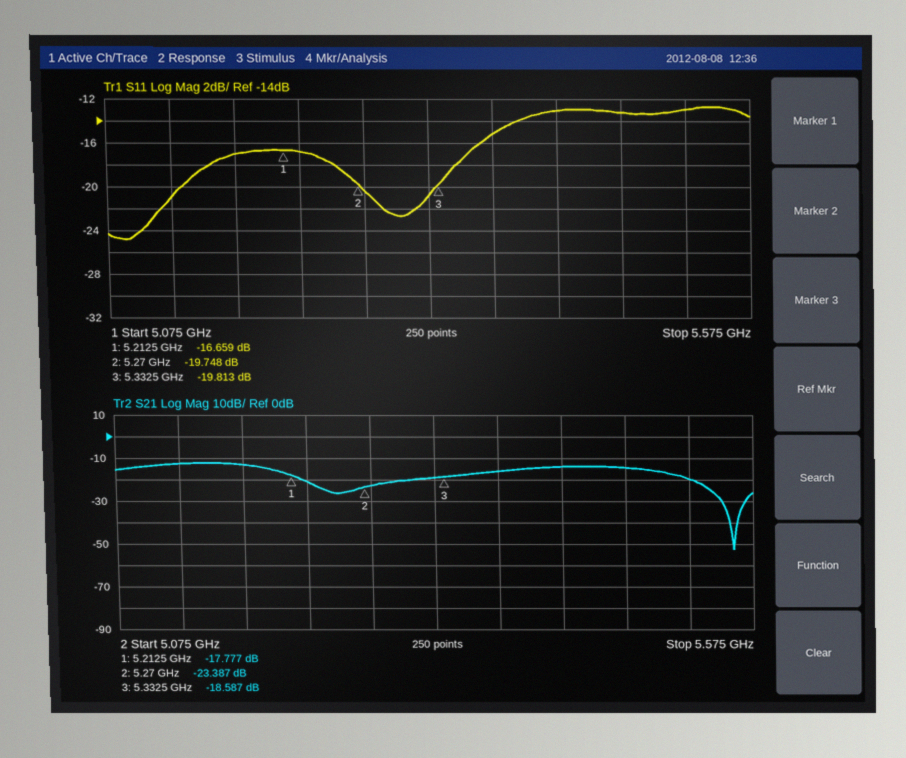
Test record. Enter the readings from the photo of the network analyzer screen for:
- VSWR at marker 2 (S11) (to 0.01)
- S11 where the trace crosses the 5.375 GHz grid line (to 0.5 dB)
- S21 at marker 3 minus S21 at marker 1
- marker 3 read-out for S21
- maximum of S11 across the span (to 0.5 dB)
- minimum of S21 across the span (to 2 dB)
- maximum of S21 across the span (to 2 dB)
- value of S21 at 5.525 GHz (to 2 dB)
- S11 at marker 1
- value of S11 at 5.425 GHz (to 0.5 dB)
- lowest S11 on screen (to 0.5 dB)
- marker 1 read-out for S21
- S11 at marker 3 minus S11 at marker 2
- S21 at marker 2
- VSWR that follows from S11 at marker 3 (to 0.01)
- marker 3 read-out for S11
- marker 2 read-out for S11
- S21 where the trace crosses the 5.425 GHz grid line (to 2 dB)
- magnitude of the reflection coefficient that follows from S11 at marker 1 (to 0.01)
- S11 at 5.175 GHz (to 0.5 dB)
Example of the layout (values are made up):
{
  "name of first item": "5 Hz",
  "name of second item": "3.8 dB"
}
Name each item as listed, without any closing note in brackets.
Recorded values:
{
  "VSWR at marker 2 (S11)": "1.23",
  "S11 where the trace crosses the 5.375 GHz grid line": "-15.0 dB",
  "S21 at marker 3 minus S21 at marker 1": "-0.810 dB",
  "marker 3 read-out for S21": "-18.587 dB",
  "maximum of S11 across the span": "-12.5 dB",
  "minimum of S21 across the span": "-52 dB",
  "maximum of S21 across the span": "-12 dB",
  "value of S21 at 5.525 GHz": "-20 dB",
  "S11 at marker 1": "-16.659 dB",
  "value of S11 at 5.425 GHz": "-13.0 dB",
  "lowest S11 on screen": "-25.0 dB",
  "marker 1 read-out for S21": "-17.777 dB",
  "S11 at marker 3 minus S11 at marker 2": "-0.065 dB",
  "S21 at marker 2": "-23.387 dB",
  "VSWR that follows from S11 at marker 3": "1.23",
  "marker 3 read-out for S11": "-19.813 dB",
  "marker 2 read-out for S11": "-19.748 dB",
  "S21 where the trace crosses the 5.425 GHz grid line": "-14 dB",
  "magnitude of the reflection coefficient that follows from S11 at marker 1": "0.15",
  "S11 at 5.175 GHz": "-17.0 dB"
}
